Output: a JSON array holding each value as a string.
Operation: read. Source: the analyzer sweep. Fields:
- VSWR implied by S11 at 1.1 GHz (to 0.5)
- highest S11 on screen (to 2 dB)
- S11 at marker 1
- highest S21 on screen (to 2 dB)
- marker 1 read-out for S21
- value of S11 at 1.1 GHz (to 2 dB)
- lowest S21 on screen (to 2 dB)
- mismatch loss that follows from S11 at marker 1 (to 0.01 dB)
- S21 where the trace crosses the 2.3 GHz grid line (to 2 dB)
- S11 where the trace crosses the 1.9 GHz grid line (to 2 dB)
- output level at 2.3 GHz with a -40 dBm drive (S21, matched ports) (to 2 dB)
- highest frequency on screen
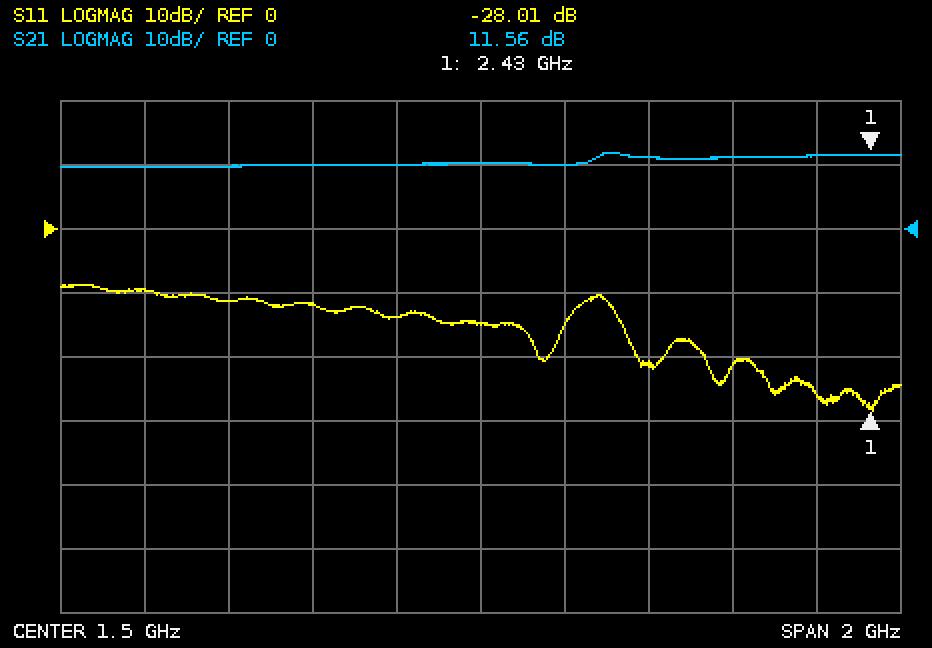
["1.5", "-8 dB", "-28.01 dB", "12 dB", "11.56 dB", "-12 dB", "10 dB", "0.01 dB", "12 dB", "-22 dB", "-28 dBm", "2.5 GHz"]
